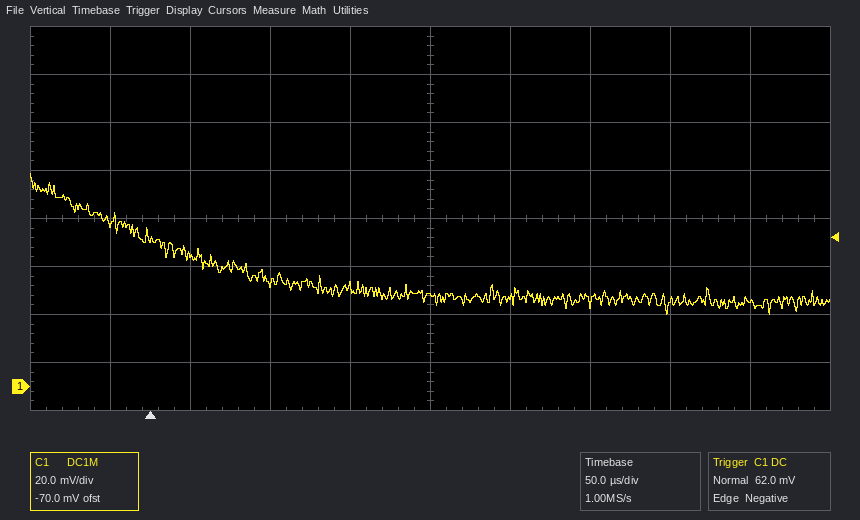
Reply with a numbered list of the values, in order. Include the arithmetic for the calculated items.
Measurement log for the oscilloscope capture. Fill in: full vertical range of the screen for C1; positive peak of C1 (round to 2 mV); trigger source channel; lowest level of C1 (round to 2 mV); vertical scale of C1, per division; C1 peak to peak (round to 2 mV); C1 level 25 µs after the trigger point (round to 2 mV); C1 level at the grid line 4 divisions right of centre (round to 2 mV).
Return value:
1. 160 mV
2. 88 mV
3. C1
4. 30 mV
5. 20 mV
6. 88 mV − (30 mV) = 58 mV
7. 54 mV
8. 36 mV
